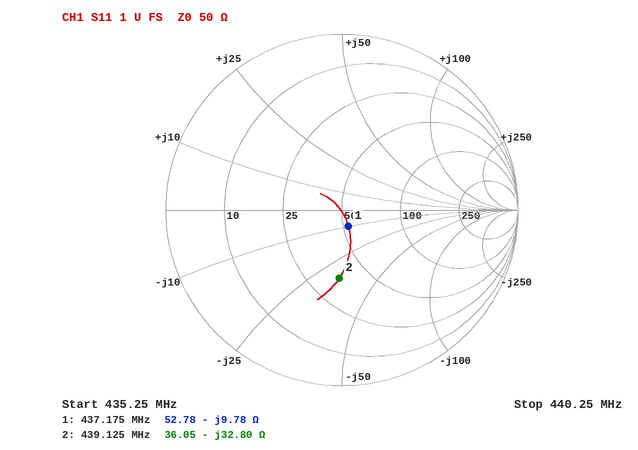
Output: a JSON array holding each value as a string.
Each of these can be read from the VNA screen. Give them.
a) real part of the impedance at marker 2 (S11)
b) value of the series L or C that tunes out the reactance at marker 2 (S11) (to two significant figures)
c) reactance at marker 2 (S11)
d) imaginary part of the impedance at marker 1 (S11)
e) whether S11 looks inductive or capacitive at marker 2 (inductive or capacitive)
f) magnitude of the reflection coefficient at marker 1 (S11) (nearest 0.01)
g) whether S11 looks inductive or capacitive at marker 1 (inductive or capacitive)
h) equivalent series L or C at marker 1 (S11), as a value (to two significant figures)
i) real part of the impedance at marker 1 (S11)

["36.05 Ω", "12 nH", "-32.80 Ω", "-9.78 Ω", "capacitive", "0.10", "capacitive", "37 pF", "52.78 Ω"]
